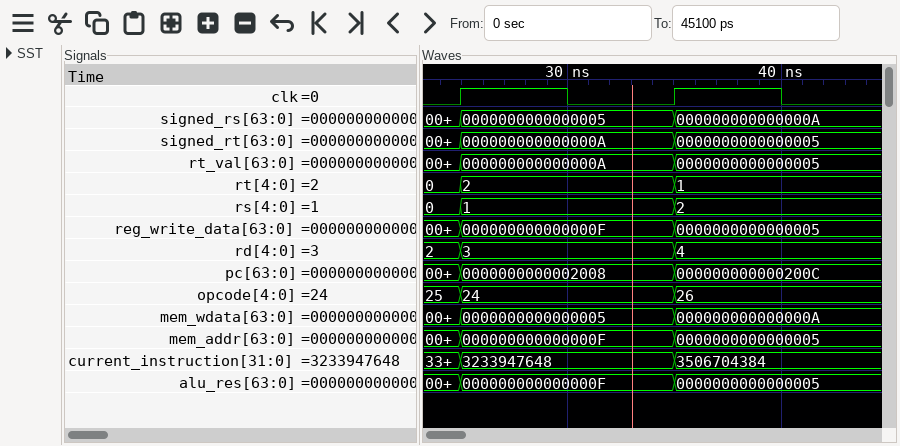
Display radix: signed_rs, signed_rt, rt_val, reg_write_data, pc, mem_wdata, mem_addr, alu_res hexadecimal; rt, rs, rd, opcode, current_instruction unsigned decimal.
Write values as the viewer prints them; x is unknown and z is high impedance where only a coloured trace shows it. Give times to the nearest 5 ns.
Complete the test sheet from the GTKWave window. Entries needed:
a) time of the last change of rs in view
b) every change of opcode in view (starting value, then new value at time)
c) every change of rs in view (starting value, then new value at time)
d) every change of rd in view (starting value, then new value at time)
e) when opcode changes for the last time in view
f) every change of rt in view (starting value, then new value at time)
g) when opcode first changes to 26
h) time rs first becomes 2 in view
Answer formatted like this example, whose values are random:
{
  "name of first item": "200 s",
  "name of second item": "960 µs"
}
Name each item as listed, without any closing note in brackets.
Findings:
{
  "time of the last change of rs in view": "35 ns",
  "every change of opcode in view": "25, 24 at 25 ns, 26 at 35 ns",
  "every change of rs in view": "0, 1 at 25 ns, 2 at 35 ns",
  "every change of rd in view": "2, 3 at 25 ns, 4 at 35 ns",
  "when opcode changes for the last time in view": "35 ns",
  "every change of rt in view": "0, 2 at 25 ns, 1 at 35 ns",
  "when opcode first changes to 26": "35 ns",
  "time rs first becomes 2 in view": "35 ns"
}
